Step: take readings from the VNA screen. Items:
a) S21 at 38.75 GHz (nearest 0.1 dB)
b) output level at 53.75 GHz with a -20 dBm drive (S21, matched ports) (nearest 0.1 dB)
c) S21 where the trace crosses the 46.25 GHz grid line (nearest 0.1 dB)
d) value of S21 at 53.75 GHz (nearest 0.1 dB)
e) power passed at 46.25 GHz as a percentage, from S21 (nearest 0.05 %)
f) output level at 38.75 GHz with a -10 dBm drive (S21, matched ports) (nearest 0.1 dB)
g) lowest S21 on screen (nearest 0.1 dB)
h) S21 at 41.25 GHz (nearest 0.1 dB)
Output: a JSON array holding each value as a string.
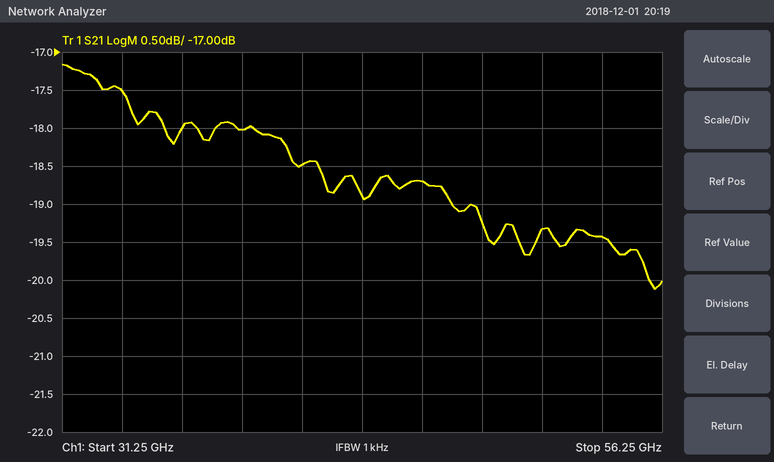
["-18.0 dB", "-39.4 dBm", "-18.7 dB", "-19.4 dB", "1.35 %", "-28.0 dBm", "-20.1 dB", "-18.5 dB"]
